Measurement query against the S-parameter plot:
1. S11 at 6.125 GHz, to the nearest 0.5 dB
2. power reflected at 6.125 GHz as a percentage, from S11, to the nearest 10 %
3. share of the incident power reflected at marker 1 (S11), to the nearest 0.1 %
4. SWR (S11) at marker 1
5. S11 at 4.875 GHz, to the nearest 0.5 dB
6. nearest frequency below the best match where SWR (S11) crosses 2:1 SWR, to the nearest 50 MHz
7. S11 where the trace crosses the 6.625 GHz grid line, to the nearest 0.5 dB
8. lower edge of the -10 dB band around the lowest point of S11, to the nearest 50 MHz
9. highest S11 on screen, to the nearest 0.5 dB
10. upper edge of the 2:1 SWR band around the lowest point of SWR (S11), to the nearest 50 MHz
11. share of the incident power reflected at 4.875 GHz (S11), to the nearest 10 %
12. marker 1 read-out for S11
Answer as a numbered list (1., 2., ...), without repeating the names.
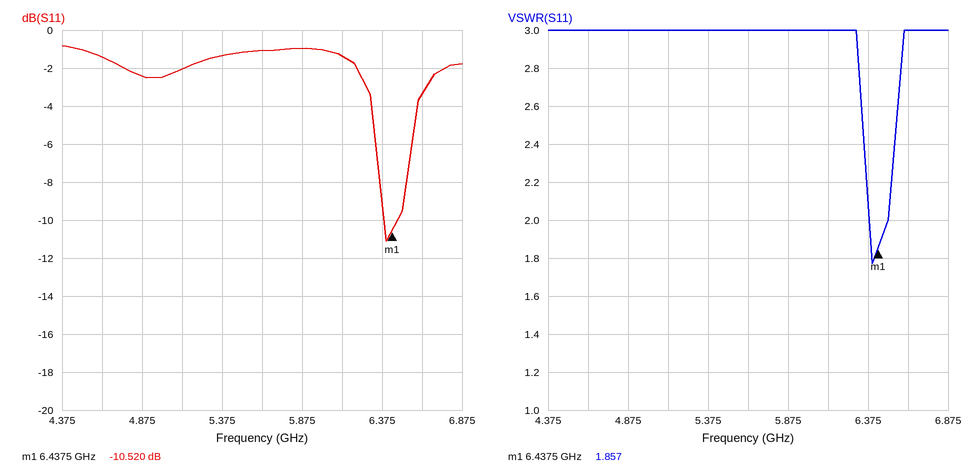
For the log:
1. -1.5 dB
2. 70 %
3. 8.9 %
4. 1.857
5. -2.5 dB
6. 6.40 GHz
7. -3.5 dB
8. 6.40 GHz
9. -1.0 dB
10. 6.50 GHz
11. 60 %
12. -10.520 dB
